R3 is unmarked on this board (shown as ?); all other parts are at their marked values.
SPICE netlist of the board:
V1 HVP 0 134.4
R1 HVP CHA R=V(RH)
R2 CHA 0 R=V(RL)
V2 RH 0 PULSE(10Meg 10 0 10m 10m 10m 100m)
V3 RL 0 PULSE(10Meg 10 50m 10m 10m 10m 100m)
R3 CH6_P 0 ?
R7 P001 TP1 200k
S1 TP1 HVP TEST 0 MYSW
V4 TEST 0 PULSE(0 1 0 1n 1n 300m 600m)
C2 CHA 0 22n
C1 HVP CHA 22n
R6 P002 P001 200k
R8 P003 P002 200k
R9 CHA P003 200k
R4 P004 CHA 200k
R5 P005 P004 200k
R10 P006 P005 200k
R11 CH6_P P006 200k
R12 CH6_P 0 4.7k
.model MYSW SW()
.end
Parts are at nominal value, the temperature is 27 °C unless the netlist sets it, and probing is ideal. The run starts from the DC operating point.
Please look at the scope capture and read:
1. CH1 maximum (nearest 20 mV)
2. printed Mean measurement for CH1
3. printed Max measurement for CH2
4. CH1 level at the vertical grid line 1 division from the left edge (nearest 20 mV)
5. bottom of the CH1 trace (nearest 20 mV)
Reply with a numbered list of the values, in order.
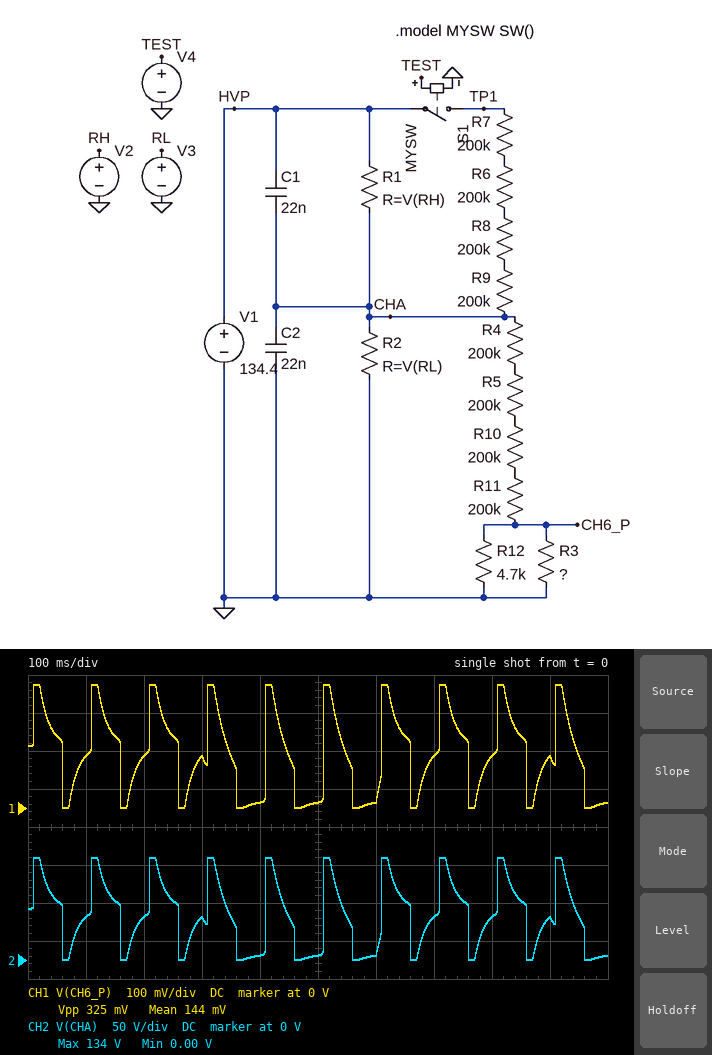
1. 320 mV
2. 144 mV
3. 134 V
4. 140 mV
5. 0 V
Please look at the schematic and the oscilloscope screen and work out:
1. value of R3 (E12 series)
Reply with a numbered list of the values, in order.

1. 3.3 kΩ
